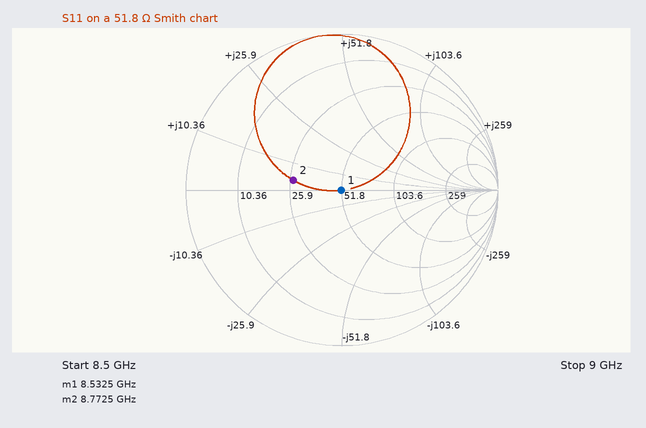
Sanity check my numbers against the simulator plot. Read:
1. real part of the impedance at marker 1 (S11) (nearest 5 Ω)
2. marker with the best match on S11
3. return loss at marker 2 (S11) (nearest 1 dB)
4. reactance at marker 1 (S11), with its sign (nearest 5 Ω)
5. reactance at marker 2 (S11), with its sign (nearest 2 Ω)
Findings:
50 Ω
marker 1
10 dB
0 Ω
+4 Ω
